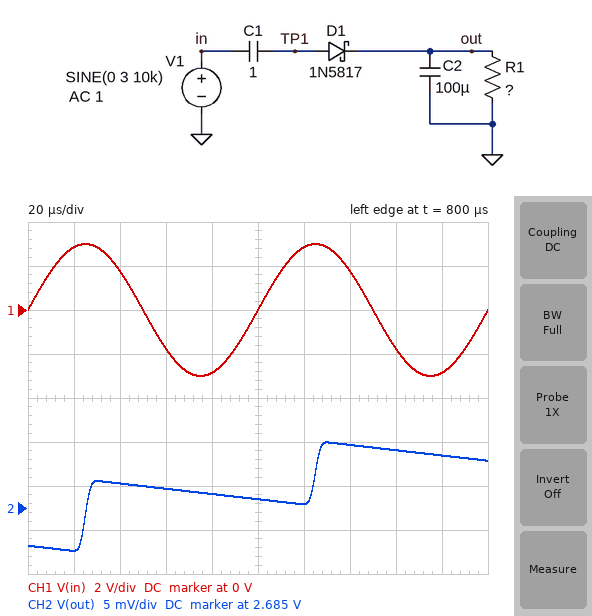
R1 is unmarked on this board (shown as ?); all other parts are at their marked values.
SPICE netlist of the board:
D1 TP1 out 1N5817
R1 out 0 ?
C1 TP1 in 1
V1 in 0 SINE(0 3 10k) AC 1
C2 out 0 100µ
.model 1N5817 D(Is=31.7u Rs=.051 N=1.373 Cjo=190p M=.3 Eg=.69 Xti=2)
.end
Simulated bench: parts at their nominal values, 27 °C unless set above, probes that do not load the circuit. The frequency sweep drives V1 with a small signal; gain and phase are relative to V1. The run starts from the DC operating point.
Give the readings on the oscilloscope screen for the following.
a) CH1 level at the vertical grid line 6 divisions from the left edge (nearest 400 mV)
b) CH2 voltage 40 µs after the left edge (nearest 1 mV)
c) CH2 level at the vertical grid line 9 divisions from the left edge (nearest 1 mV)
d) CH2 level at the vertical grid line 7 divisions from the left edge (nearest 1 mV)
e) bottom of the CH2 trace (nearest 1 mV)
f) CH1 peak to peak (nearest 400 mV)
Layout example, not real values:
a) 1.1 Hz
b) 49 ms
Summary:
a) 2.8 V
b) 2.688 V
c) 2.691 V
d) 2.692 V
e) 2.680 V
f) 6.0 V
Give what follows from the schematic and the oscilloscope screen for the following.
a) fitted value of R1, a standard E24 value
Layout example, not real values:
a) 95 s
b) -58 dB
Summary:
a) 910 Ω
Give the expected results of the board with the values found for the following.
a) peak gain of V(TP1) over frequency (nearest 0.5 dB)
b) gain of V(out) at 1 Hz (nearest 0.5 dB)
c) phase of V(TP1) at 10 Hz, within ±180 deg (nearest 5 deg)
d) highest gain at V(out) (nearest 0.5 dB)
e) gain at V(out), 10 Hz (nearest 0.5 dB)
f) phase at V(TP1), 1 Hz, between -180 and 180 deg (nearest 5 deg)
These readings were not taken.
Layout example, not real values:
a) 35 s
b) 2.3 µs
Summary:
a) 0 dB
b) -7.5 dB
c) 0 deg
d) -7.0 dB
e) -17.5 dB
f) 0 deg
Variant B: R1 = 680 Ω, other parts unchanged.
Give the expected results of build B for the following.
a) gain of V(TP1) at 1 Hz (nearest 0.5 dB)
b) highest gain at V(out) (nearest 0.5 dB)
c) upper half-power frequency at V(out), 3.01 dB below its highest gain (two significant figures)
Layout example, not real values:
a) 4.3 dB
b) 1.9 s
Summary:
a) 0 dB
b) -8.5 dB
c) 3.8 Hz
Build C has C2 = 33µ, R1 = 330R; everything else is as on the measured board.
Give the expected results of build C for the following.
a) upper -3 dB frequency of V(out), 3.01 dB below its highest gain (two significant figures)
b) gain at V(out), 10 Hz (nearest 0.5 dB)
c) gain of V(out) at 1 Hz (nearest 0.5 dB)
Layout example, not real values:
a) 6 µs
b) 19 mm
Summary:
a) 19 Hz
b) -14.0 dB
c) -13.0 dB
